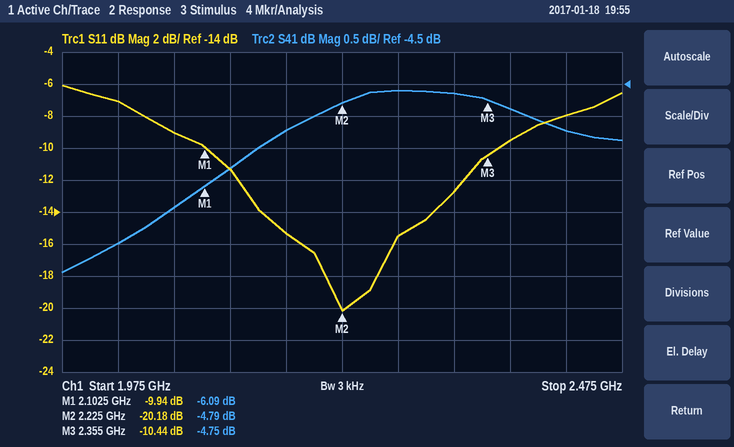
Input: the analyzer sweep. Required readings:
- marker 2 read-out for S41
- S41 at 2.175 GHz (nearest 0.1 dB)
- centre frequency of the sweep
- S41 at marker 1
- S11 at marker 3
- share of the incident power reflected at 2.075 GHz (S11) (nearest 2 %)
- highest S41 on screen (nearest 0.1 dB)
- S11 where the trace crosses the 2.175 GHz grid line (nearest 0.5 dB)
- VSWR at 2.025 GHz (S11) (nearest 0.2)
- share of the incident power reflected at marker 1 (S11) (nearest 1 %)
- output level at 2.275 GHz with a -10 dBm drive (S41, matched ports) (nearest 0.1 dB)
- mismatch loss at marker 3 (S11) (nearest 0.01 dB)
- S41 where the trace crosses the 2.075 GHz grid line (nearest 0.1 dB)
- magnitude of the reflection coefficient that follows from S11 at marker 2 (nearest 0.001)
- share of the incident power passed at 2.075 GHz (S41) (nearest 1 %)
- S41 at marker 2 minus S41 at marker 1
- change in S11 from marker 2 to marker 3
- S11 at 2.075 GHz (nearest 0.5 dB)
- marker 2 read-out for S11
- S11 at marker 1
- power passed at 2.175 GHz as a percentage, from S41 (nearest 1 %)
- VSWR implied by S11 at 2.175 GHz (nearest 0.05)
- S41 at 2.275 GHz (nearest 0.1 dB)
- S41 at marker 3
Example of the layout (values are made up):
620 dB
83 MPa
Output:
-4.79 dB
-5.2 dB
2.225 GHz
-6.09 dB
-10.44 dB
12 %
-4.6 dB
-15.5 dB
2.6
10 %
-14.6 dBm
0.41 dB
-6.4 dB
0.098
23 %
1.30 dB
9.74 dB
-9.0 dB
-20.18 dB
-9.94 dB
30 %
1.40
-4.6 dB
-4.75 dB
